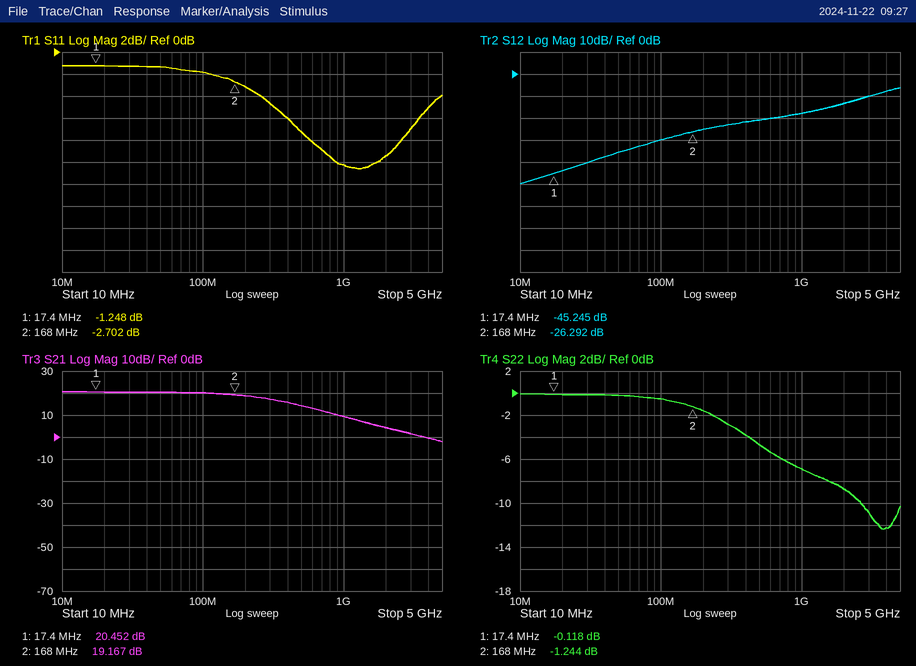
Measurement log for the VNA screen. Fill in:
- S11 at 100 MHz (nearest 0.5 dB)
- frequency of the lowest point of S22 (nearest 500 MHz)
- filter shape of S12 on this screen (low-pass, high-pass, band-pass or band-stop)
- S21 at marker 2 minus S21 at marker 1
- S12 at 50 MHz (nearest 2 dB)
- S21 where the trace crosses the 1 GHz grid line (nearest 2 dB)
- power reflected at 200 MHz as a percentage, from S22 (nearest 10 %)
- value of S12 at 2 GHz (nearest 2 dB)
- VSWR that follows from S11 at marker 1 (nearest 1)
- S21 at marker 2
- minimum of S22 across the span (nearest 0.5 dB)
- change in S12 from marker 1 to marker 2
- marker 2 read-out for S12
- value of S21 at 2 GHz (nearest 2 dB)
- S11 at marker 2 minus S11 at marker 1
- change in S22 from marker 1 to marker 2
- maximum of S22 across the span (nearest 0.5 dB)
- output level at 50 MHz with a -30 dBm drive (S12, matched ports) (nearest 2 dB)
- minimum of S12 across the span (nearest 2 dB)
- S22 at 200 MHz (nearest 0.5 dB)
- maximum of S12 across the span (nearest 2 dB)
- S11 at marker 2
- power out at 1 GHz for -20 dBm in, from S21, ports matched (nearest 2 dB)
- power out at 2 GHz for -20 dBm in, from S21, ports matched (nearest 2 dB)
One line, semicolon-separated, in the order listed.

-2.0 dB; 4.0 GHz; high-pass; -1.285 dB; -36 dB; 10 dB; 70 %; -14 dB; 14; 19.167 dB; -12.5 dB; 18.953 dB; -26.292 dB; 4 dB; -1.454 dB; -1.126 dB; 0.0 dB; -66 dBm; -50 dB; -1.5 dB; -6 dB; -2.702 dB; -10 dBm; -16 dBm
